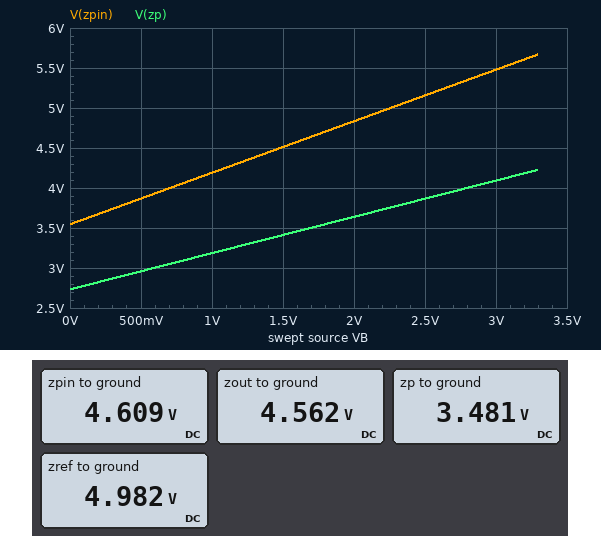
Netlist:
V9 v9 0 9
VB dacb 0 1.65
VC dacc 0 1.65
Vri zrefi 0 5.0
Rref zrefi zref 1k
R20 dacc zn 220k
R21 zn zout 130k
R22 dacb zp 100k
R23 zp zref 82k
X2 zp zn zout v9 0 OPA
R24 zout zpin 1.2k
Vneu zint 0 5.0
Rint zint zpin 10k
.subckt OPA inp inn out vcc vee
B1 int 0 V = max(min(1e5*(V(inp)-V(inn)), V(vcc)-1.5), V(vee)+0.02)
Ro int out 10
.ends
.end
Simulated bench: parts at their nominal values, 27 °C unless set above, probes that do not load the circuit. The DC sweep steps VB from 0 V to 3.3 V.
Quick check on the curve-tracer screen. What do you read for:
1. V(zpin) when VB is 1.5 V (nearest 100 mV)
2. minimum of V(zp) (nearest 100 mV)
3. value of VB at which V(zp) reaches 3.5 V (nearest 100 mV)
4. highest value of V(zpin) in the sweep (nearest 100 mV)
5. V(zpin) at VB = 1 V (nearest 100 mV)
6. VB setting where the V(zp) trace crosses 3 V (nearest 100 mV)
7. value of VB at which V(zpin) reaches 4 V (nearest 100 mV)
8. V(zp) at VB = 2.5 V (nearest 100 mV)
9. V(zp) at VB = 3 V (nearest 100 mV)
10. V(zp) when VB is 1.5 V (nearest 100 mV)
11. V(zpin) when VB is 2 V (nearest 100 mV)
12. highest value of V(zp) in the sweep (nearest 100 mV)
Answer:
4.5 V
2.7 V
1.7 V
5.7 V
4.2 V
600 mV
700 mV
3.9 V
4.1 V
3.4 V
4.8 V
4.2 V
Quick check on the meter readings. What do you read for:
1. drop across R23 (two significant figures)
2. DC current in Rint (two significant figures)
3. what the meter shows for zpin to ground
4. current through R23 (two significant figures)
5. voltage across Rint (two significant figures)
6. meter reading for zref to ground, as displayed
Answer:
1.5 V
39 µA
4.609 V
18 µA
390 mV
4.982 V
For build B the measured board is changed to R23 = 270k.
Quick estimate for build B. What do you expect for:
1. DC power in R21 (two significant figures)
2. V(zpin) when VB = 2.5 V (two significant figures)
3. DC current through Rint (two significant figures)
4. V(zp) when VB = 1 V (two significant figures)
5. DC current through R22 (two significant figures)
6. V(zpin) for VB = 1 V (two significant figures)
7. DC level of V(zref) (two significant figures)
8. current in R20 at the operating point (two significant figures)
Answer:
2.2 µW
4.2 V
170 µA
2.1 V
9.0 µA
2.6 V
5.0 V
4.1 µA
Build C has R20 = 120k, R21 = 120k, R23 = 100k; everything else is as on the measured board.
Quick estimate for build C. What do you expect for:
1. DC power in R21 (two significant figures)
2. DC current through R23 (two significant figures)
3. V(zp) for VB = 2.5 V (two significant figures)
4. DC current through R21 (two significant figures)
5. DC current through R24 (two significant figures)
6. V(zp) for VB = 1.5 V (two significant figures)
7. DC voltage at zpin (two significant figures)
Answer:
23 µW
17 µA
3.7 V
14 µA
1.5 µA
3.2 V
5.0 V
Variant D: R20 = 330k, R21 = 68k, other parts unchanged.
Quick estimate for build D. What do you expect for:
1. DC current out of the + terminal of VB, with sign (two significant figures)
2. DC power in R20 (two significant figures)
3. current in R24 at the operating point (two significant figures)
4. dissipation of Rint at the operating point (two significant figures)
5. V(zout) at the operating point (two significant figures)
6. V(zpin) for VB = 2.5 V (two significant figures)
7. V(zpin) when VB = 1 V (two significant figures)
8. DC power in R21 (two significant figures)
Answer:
-18 µA
10 µW
100 µA
100 µW
3.9 V
4.4 V
3.7 V
2.1 µW
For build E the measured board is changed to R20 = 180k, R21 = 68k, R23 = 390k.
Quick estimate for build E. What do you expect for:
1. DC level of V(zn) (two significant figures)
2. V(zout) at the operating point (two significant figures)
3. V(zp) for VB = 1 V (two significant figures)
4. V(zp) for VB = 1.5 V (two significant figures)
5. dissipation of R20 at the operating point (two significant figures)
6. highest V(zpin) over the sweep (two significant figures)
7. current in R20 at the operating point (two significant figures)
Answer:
2.3 V
2.6 V
1.8 V
2.2 V
2.6 µW
4.5 V
3.8 µA
